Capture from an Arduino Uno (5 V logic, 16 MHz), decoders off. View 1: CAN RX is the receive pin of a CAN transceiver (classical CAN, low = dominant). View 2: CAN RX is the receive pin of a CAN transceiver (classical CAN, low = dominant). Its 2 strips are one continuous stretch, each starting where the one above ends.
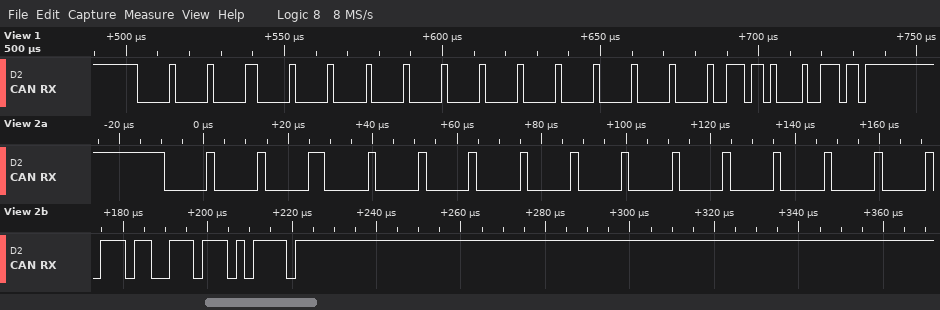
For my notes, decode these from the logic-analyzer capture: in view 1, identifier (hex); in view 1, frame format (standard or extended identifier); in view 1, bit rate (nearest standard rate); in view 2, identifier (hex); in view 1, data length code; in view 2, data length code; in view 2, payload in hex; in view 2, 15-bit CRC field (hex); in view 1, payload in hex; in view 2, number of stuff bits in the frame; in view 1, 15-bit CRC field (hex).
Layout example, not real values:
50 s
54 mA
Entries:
0x000
standard
500 kbit/s
0x000
8
8
00 00 00 00 00 00 00 3B
0x1DD7
00 00 00 00 00 00 00 1D
15
0x509D
